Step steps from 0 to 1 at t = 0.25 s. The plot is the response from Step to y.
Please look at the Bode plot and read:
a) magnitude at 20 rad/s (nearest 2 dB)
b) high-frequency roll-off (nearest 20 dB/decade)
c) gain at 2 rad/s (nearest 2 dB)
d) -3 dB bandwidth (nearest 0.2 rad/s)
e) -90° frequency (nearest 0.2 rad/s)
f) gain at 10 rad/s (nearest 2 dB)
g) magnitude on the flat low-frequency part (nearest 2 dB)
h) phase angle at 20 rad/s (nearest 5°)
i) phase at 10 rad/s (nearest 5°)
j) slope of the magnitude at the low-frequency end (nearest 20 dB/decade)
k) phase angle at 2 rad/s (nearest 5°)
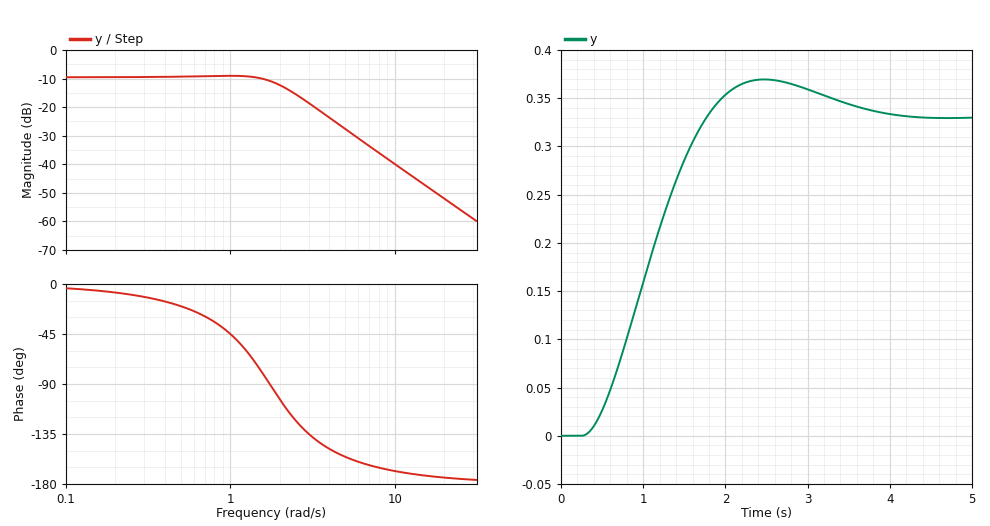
-52 dB
-40 dB/decade
-12 dB
2.0 rad/s
1.8 rad/s
-40 dB
-10 dB
-175°
-170°
0 dB/decade
-105°
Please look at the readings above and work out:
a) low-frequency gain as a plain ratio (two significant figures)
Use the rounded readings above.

0.32
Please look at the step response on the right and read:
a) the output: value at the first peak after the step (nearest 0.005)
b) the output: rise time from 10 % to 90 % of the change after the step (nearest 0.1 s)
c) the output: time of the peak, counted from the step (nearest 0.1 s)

0.370
1.0 s
2.2 s
